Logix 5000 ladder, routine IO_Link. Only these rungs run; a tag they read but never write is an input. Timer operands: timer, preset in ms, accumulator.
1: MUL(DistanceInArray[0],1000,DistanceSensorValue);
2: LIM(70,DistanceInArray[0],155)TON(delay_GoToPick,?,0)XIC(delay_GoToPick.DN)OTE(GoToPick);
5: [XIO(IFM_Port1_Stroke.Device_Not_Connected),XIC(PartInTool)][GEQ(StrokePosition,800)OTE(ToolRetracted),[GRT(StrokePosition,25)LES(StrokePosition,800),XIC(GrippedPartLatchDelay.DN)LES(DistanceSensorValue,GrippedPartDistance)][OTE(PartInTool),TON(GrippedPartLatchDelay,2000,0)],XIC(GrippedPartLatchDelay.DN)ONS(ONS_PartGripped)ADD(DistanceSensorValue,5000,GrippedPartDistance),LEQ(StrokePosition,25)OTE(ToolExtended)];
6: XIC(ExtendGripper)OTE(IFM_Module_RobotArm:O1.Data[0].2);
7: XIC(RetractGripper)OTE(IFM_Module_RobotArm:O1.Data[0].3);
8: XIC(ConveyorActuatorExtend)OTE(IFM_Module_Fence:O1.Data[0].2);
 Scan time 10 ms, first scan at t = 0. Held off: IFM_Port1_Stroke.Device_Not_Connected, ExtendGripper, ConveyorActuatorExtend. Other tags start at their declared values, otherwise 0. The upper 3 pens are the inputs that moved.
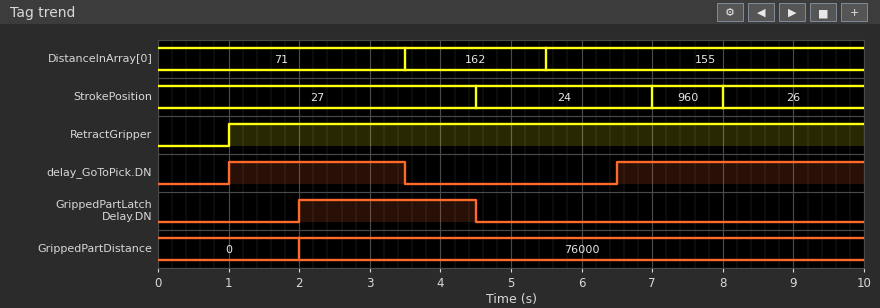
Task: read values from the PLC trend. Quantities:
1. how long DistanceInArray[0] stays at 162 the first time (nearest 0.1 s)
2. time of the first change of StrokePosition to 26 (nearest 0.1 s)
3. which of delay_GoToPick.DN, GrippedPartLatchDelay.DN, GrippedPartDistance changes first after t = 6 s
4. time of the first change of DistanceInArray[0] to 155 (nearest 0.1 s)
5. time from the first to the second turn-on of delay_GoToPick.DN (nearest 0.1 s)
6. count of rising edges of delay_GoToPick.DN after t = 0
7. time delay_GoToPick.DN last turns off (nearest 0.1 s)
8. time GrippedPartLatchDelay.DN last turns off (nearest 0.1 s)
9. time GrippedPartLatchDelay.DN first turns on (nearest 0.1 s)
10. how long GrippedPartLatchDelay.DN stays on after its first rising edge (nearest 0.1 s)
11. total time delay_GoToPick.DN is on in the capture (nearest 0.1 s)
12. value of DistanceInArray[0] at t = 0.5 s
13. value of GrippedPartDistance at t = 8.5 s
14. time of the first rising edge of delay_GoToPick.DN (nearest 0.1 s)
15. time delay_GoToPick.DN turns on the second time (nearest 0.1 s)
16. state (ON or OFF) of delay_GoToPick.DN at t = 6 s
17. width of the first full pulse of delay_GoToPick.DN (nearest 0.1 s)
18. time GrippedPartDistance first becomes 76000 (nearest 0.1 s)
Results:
2.0 s
8.0 s
delay_GoToPick.DN
5.5 s
5.5 s
2
3.5 s
4.5 s
2.0 s
2.5 s
6.0 s
71
76000
1.0 s
6.5 s
OFF
2.5 s
2.0 s
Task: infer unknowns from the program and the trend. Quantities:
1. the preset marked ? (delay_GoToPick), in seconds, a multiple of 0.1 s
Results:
1.0 s
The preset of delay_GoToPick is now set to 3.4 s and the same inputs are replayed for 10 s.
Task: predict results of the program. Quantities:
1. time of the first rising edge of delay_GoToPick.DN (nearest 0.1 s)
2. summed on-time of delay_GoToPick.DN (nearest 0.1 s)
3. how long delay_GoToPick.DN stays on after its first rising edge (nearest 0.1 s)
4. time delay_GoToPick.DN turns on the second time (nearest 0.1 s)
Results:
3.4 s
1.2 s
0.1 s
8.9 s
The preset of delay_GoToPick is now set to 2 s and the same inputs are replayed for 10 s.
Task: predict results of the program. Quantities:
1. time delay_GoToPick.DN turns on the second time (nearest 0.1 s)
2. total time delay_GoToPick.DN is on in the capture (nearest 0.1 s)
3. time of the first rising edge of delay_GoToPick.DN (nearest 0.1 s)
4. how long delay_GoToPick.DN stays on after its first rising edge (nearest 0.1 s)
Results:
7.5 s
4.0 s
2.0 s
1.5 s
